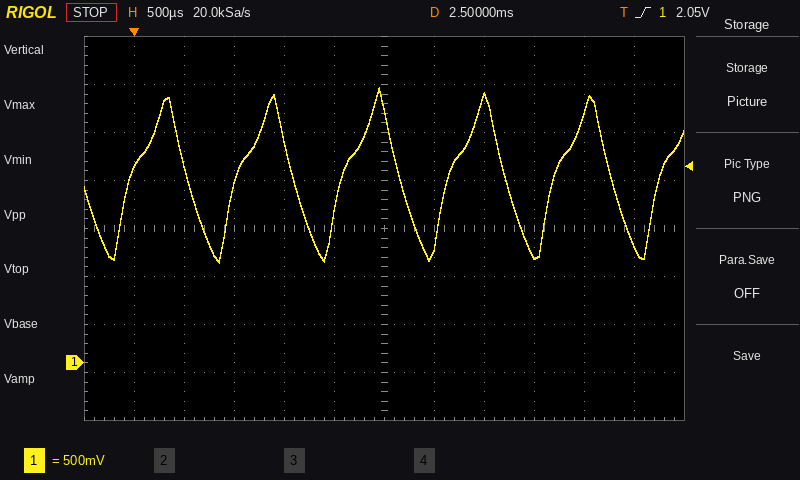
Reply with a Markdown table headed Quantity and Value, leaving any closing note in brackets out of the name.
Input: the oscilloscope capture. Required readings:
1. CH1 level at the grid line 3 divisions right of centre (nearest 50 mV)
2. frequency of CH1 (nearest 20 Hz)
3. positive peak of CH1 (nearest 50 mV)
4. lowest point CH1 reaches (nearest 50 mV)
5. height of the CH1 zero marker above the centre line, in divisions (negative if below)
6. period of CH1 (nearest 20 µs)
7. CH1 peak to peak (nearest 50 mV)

| Quantity | Value |
|---|---|
| CH1 level at the grid line 3 divisions right of centre | 1.10 V |
| frequency of CH1 | 940 Hz |
| positive peak of CH1 | 2.85 V |
| lowest point CH1 reaches | 1.05 V |
| height of the CH1 zero marker above the centre line, in divisions | -2.8 div |
| period of CH1 | 1.06 ms |
| CH1 peak to peak | 1.80 V |
